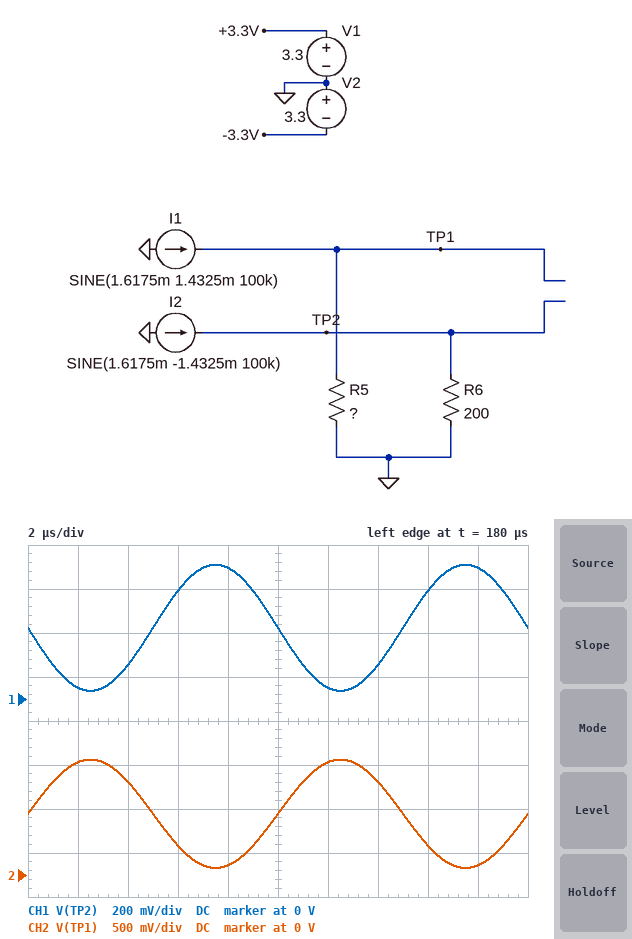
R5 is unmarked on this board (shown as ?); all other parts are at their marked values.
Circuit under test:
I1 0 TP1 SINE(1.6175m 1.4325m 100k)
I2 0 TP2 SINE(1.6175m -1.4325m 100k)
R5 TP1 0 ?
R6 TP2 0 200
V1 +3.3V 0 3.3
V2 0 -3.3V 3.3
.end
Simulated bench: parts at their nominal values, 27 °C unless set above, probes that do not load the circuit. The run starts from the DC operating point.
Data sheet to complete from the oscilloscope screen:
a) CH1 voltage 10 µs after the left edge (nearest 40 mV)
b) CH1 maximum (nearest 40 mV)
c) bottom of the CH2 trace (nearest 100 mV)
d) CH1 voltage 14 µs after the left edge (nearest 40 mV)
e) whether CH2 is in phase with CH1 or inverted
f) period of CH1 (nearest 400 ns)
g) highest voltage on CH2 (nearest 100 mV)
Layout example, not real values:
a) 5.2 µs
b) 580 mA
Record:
a) 320 mV
b) 600 mV
c) 100 mV
d) 160 mV
e) inverted
f) 10.0 µs
g) 1.3 V
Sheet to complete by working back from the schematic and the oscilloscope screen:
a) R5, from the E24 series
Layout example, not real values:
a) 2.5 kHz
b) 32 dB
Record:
a) 430 Ω
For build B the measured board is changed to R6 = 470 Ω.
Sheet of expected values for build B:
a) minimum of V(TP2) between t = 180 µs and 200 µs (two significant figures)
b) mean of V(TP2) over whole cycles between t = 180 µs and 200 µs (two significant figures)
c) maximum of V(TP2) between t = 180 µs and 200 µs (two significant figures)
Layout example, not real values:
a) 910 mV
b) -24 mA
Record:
a) 87 mV
b) 760 mV
c) 1.4 V
